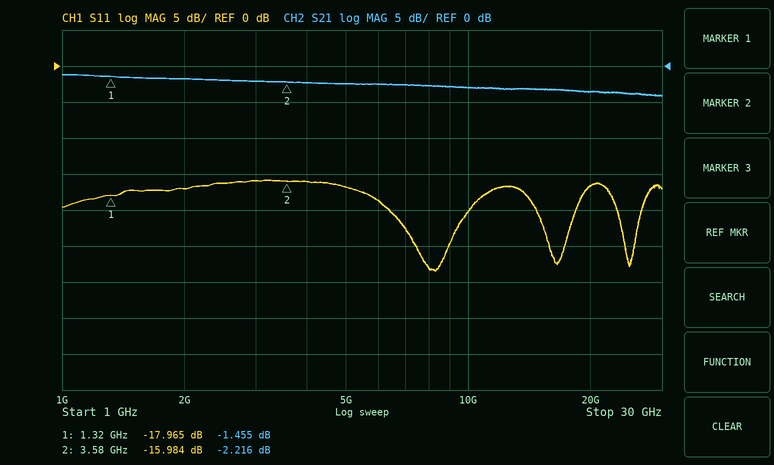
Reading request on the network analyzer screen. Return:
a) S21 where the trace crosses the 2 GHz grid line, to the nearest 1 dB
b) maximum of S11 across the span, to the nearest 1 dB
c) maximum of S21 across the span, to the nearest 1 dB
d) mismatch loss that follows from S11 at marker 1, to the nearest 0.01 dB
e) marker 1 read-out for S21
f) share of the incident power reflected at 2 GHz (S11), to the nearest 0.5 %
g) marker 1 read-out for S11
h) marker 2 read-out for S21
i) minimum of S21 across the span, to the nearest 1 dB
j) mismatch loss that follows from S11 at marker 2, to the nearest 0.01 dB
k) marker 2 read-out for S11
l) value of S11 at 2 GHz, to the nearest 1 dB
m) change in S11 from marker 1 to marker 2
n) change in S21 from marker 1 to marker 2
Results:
-2 dB
-16 dB
-1 dB
0.07 dB
-1.455 dB
2.0 %
-17.965 dB
-2.216 dB
-4 dB
0.11 dB
-15.984 dB
-17 dB
1.981 dB
-0.761 dB
